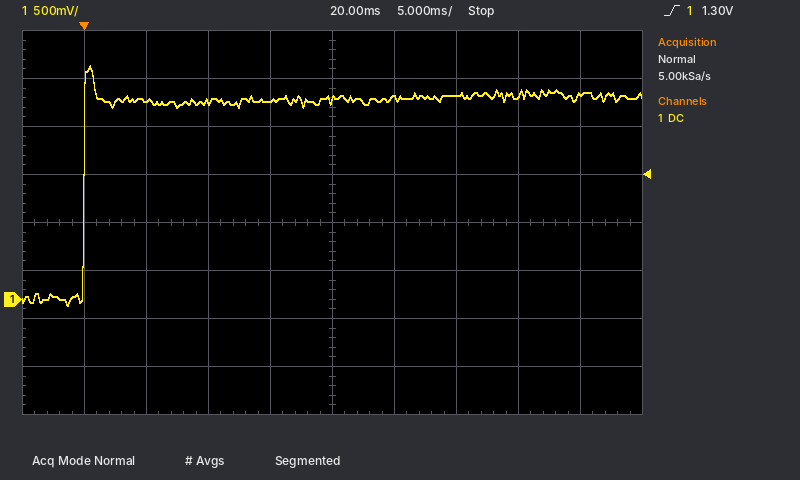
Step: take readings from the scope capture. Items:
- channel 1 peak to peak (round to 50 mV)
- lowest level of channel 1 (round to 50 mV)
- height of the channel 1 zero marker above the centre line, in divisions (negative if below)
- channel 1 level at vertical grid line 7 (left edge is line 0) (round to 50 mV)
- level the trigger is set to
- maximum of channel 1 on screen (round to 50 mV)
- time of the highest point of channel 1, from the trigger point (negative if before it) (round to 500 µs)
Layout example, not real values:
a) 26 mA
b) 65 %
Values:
a) 2.50 V
b) -50 mV
c) -1.6 div
d) 2.10 V
e) 1.30 V
f) 2.45 V
g) +500 µs
